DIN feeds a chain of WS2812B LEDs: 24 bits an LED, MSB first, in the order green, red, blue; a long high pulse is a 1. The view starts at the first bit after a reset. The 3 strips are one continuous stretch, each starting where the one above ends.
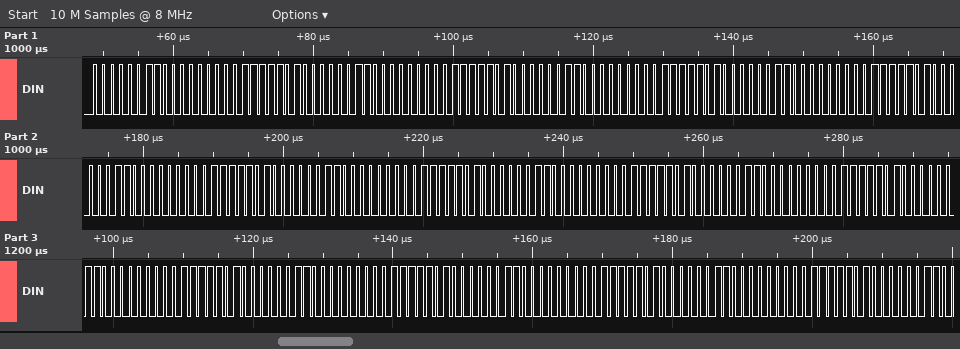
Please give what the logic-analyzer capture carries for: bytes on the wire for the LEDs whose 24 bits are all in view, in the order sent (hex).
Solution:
03 00 7D 03 00 7D 03 00 7D 03 00 7D 03 00 7D 03 00 7D 03 00 7D 03 00 7D 03 00 7D 03 00 7D 03 00 7D 03 00 7D
